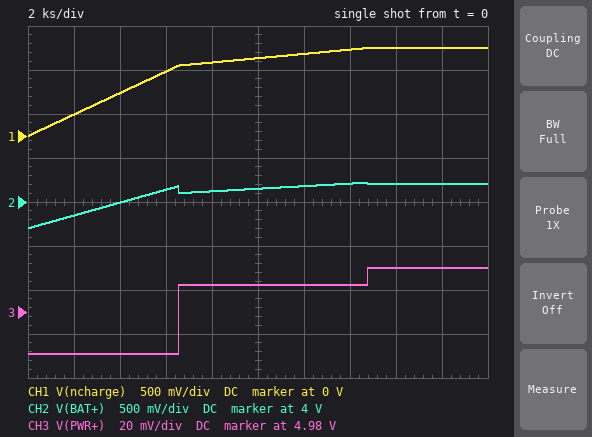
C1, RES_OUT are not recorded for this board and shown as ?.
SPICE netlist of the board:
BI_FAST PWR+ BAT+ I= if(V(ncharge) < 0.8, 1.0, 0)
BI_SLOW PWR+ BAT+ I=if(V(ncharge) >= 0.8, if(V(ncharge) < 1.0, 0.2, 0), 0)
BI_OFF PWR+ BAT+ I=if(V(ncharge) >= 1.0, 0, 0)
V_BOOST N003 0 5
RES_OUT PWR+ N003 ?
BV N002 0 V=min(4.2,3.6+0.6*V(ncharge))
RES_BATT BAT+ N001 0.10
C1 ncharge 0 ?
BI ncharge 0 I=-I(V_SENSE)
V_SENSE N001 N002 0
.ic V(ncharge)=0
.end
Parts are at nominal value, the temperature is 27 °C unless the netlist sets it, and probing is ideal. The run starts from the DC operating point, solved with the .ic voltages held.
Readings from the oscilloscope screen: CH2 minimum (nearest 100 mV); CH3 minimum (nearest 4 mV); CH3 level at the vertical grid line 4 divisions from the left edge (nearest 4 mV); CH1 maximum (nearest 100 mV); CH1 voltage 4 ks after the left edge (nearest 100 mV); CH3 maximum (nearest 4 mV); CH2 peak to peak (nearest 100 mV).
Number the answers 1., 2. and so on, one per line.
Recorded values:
1. 3.7 V
2. 4.960 V
3. 4.992 V
4. 1.0 V
5. 500 mV
6. 5.000 V
7. 500 mV
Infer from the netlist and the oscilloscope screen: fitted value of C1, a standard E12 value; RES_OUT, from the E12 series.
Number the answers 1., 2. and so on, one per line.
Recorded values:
1. 8.2 kF
2. 0.039 Ω
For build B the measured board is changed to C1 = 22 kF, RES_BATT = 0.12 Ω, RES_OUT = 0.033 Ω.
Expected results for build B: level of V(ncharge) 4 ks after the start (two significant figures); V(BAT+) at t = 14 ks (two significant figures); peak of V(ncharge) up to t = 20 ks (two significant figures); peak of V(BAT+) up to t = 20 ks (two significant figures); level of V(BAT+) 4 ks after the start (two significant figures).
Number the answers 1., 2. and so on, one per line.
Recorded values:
1. 180 mV
2. 4.1 V
3. 820 mV
4. 4.2 V
5. 3.8 V
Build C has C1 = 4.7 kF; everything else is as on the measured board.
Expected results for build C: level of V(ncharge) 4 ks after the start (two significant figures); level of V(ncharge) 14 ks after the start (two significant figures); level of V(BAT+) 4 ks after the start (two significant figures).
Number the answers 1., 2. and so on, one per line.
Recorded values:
1. 810 mV
2. 1.0 V
3. 4.1 V
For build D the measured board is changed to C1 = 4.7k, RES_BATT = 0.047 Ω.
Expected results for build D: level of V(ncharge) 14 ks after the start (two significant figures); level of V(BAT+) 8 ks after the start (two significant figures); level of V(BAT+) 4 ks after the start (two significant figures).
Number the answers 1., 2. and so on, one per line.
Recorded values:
1. 1.0 V
2. 4.2 V
3. 4.1 V
